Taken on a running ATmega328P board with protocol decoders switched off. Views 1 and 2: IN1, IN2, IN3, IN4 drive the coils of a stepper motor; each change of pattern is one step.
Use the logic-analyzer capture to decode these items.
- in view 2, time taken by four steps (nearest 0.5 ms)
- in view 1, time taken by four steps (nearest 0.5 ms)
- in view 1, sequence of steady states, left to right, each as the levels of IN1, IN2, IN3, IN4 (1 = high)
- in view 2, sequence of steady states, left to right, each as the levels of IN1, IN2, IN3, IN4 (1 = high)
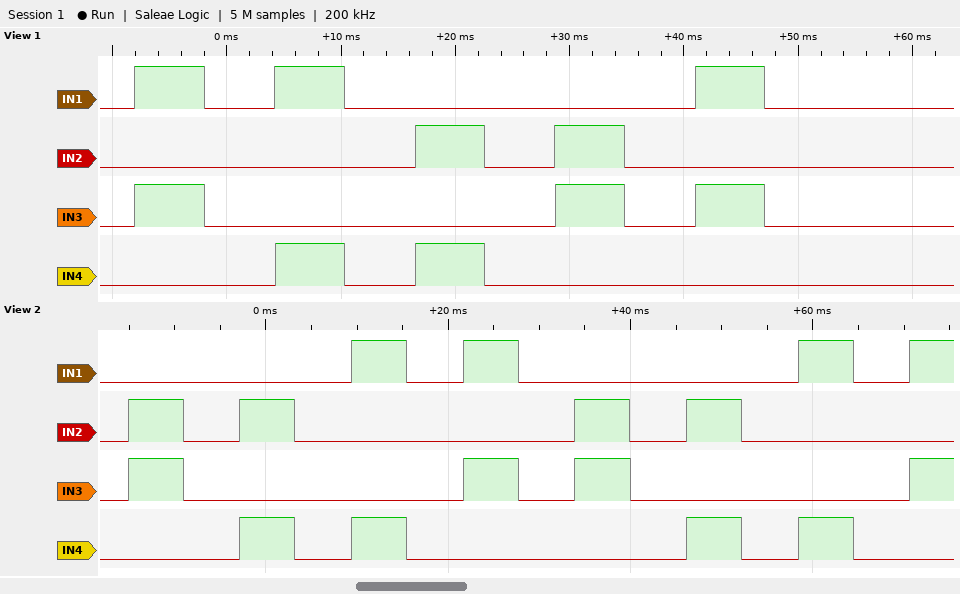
24.5 ms
24.5 ms
0000 1010 0000 1001 0000 0101 0000 0110 0000 1010 0000
0000 0110 0000 0101 0000 1001 0000 1010 0000 0110 0000 0101 0000 1001 0000 1010
